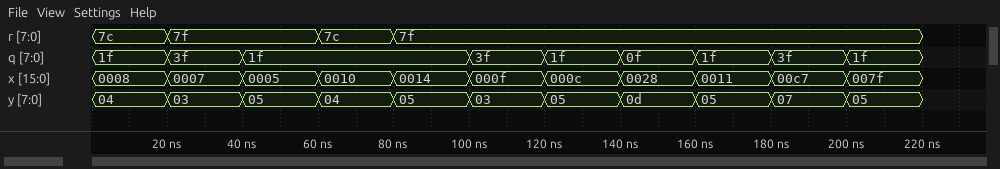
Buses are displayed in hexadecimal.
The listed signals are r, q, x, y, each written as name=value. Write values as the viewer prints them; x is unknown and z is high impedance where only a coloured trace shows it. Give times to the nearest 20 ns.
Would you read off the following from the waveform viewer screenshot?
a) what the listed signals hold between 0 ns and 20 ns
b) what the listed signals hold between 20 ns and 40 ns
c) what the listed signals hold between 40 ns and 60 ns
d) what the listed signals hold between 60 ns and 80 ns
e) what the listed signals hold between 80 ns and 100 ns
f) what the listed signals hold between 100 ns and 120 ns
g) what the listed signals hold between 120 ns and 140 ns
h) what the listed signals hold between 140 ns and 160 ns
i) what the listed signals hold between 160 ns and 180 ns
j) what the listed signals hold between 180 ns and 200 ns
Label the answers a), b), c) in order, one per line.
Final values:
a) r=7c, q=1f, x=0008, y=04
b) r=7f, q=3f, x=0007, y=03
c) r=7f, q=1f, x=0005, y=05
d) r=7c, q=1f, x=0010, y=04
e) r=7f, q=1f, x=0014, y=05
f) r=7f, q=3f, x=000f, y=03
g) r=7f, q=1f, x=000c, y=05
h) r=7f, q=0f, x=0028, y=0d
i) r=7f, q=1f, x=0011, y=05
j) r=7f, q=3f, x=00c7, y=07
